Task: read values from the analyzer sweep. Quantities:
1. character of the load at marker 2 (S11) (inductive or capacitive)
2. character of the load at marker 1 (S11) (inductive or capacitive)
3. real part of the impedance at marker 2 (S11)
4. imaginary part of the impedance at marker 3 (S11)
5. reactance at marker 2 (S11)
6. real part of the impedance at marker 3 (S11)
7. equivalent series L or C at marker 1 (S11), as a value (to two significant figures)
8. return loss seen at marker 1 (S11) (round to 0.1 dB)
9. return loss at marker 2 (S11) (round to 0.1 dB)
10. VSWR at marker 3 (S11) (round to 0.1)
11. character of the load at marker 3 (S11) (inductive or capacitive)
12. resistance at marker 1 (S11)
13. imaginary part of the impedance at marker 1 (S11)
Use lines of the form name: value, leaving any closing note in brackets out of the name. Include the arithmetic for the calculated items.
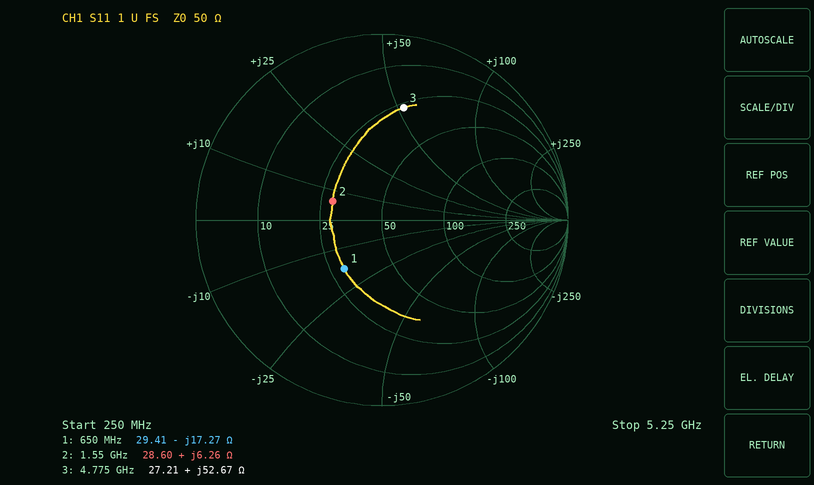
character of the load at marker 2 (S11): inductive
character of the load at marker 1 (S11): capacitive
real part of the impedance at marker 2: 28.60 Ω
imaginary part of the impedance at marker 3: +52.67 Ω
reactance at marker 2: +6.26 Ω
real part of the impedance at marker 3: 27.21 Ω
equivalent series L or C at marker 1 (S11), as a value: C = 1/(2π × 650 MHz × 17.27 Ω) ≈ 14 pF
return loss seen at marker 1 (S11): 9.6 dB
return loss at marker 2 (S11): 11.0 dB
VSWR at marker 3 (S11): 4.2
character of the load at marker 3 (S11): inductive
resistance at marker 1: 29.41 Ω
imaginary part of the impedance at marker 1: -17.27 Ω
